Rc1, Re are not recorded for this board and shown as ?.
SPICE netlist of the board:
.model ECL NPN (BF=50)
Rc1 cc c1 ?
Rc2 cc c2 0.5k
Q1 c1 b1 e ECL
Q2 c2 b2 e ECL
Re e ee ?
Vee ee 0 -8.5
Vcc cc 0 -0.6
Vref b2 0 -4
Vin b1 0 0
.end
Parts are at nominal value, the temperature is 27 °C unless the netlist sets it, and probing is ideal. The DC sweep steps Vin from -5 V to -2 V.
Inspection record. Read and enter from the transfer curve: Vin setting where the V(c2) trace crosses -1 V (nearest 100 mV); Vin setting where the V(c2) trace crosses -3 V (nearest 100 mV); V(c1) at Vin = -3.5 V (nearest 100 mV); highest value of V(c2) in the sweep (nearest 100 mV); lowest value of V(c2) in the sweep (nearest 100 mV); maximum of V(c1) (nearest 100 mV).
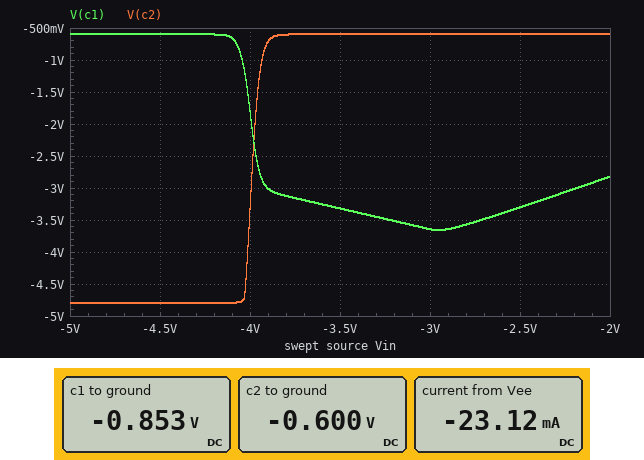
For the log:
-3.9 V
-4.0 V
-3.3 V
-600 mV
-4.8 V
-600 mV
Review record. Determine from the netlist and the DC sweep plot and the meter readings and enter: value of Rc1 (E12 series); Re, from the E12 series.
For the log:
220 Ω
330 Ω
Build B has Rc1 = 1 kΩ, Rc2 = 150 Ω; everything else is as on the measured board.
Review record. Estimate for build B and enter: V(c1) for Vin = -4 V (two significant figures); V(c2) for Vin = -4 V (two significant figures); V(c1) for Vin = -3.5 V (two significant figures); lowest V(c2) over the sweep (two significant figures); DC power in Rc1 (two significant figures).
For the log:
-4.8 V
-1.5 V
-4.3 V
-2.2 V
65 µW
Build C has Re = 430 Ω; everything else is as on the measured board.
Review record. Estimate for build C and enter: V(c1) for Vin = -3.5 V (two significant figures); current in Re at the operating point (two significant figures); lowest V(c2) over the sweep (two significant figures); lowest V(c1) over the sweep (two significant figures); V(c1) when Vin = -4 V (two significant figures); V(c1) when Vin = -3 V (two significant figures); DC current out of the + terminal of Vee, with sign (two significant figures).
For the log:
-2.7 V
18 mA
-4.7 V
-3.2 V
-1.5 V
-2.9 V
-18 mA
